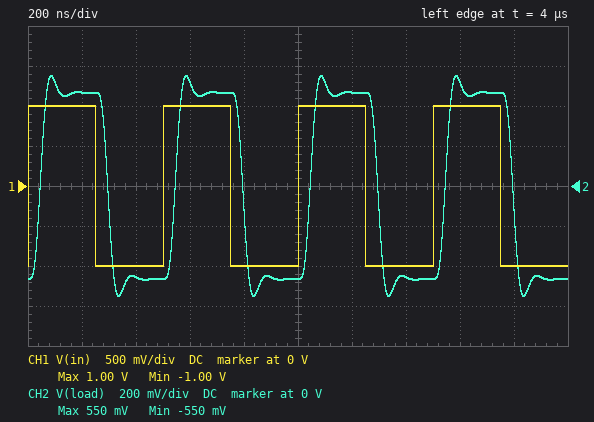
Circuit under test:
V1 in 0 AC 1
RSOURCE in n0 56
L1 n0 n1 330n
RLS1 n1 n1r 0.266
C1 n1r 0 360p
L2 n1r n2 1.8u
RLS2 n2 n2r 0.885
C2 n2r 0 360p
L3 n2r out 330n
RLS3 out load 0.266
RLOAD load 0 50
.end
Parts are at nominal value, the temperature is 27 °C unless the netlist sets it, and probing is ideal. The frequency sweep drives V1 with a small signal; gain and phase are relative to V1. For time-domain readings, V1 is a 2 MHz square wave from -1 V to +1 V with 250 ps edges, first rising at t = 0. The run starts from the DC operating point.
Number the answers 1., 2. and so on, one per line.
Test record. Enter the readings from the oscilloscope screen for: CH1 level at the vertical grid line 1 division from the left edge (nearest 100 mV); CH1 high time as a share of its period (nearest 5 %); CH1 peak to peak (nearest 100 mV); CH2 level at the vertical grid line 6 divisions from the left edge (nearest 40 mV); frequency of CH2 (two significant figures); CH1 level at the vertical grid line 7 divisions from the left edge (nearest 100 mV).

1. 1.0 V
2. 50 %
3. 2.0 V
4. 480 mV
5. 2.0 MHz
6. -1.0 V
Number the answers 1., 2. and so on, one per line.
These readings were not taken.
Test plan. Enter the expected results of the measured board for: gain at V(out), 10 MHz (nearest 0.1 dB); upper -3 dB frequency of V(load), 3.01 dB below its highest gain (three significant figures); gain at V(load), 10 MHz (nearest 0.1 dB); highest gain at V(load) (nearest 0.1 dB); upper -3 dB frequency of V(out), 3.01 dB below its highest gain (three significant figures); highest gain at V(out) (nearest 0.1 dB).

1. -8.9 dB
2. 10.6 MHz
3. -9.0 dB
4. -6.6 dB
5. 10.6 MHz
6. -6.6 dB
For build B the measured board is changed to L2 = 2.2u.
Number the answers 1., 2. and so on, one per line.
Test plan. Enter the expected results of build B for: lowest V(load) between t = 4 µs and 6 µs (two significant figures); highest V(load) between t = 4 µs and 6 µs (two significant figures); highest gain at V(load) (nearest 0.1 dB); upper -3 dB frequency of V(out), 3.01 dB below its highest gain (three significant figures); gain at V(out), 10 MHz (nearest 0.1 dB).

1. -530 mV
2. 530 mV
3. -6.6 dB
4. 9.18 MHz
5. -10.7 dB
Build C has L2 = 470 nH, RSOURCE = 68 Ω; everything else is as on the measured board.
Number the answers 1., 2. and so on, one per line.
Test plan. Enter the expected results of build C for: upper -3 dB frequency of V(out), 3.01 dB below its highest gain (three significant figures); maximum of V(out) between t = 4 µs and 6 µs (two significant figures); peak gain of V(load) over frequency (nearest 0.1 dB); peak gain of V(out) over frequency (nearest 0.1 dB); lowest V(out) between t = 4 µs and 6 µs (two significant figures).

1. 20.7 MHz
2. 480 mV
3. -7.6 dB
4. -7.5 dB
5. -480 mV
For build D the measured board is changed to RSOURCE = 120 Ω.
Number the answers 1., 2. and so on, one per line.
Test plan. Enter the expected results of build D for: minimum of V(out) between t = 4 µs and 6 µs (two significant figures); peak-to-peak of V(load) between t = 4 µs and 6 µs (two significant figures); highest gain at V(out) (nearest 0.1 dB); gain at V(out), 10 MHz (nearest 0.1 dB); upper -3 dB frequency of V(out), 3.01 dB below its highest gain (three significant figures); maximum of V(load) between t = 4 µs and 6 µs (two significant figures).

1. -380 mV
2. 760 mV
3. -10.0 dB
4. -13.0 dB
5. 10.0 MHz
6. 380 mV
